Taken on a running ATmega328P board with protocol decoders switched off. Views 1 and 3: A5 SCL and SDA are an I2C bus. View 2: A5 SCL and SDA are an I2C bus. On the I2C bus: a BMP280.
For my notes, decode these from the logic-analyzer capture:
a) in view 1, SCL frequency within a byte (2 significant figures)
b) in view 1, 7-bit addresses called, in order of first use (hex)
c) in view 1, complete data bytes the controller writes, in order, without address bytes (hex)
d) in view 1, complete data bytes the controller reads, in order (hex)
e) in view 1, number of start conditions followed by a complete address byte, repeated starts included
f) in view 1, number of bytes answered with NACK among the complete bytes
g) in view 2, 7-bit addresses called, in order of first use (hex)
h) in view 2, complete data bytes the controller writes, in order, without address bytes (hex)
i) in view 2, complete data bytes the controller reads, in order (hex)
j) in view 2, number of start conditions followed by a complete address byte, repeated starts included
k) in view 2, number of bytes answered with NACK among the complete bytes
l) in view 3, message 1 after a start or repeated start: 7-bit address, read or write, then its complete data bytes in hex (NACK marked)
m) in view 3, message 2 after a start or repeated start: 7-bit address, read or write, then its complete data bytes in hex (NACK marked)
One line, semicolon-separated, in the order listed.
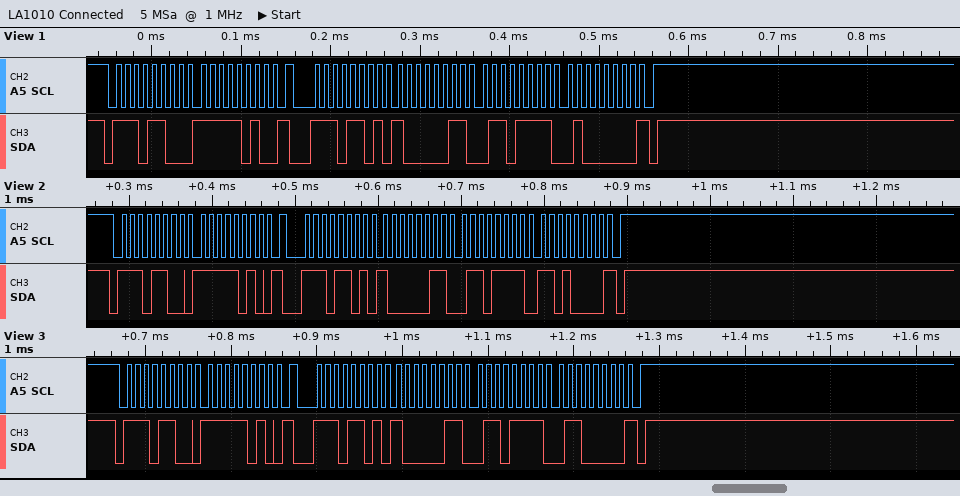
100 kHz; 0x76; FA; 83 6F 40; 2; 1; 0x76; FA; 83 6F D0; 2; 1; 0x76 write: FA; 0x76 read: 83 6F 60 NACK
